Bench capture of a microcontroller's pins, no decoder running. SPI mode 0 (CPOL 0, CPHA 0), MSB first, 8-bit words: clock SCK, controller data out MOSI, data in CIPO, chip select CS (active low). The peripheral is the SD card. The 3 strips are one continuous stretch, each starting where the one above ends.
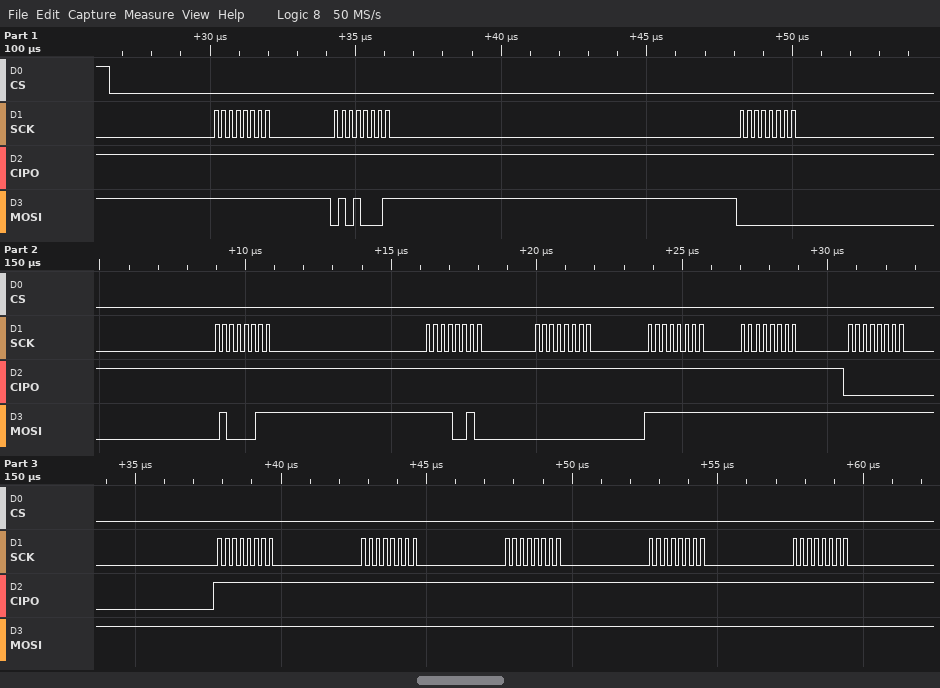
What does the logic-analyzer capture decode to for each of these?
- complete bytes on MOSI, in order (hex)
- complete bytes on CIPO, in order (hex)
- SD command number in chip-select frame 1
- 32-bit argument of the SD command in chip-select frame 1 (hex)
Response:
0xFF 0x51 0x00 0x43 0xF2 0x00 0xFF 0xFF 0xFF 0xFF 0xFF 0xFF 0xFF 0xFF
0xFF 0xFF 0xFF 0xFF 0xFF 0xFF 0xFF 0xFF 0x00 0xFF 0xFF 0xFF 0xFF 0xFF
CMD17
0x0043F200
